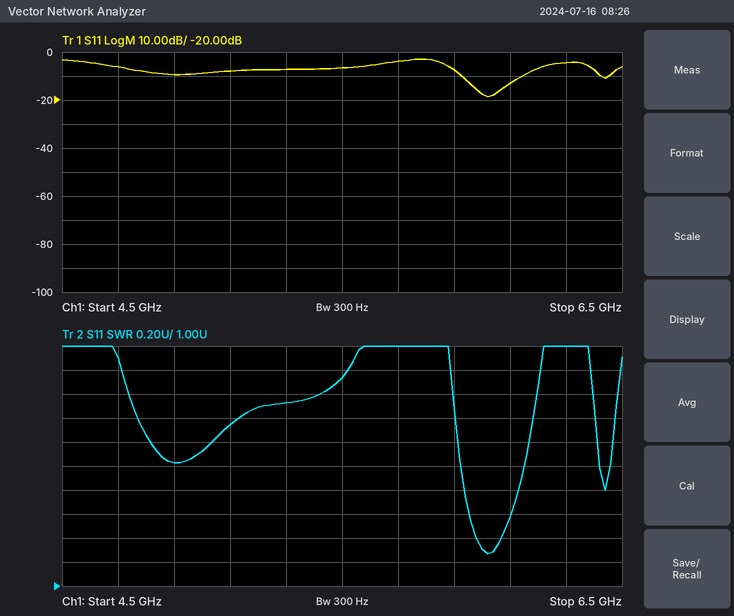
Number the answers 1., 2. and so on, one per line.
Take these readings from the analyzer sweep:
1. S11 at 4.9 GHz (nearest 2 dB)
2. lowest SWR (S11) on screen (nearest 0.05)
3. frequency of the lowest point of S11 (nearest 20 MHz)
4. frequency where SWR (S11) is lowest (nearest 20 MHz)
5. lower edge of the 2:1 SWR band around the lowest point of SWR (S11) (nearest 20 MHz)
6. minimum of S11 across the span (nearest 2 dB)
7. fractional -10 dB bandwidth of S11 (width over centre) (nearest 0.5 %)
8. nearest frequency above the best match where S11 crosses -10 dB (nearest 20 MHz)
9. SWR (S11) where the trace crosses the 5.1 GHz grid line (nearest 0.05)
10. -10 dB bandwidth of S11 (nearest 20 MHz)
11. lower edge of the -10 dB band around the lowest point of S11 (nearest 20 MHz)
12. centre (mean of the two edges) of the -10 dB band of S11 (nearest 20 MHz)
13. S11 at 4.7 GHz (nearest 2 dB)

1. -10 dB
2. 1.25
3. 6.02 GHz
4. 6.02 GHz
5. 5.92 GHz
6. -18 dB
7. 3.5 %
8. 6.14 GHz
9. 2.35
10. 220 MHz
11. 5.92 GHz
12. 6.04 GHz
13. -6 dB
